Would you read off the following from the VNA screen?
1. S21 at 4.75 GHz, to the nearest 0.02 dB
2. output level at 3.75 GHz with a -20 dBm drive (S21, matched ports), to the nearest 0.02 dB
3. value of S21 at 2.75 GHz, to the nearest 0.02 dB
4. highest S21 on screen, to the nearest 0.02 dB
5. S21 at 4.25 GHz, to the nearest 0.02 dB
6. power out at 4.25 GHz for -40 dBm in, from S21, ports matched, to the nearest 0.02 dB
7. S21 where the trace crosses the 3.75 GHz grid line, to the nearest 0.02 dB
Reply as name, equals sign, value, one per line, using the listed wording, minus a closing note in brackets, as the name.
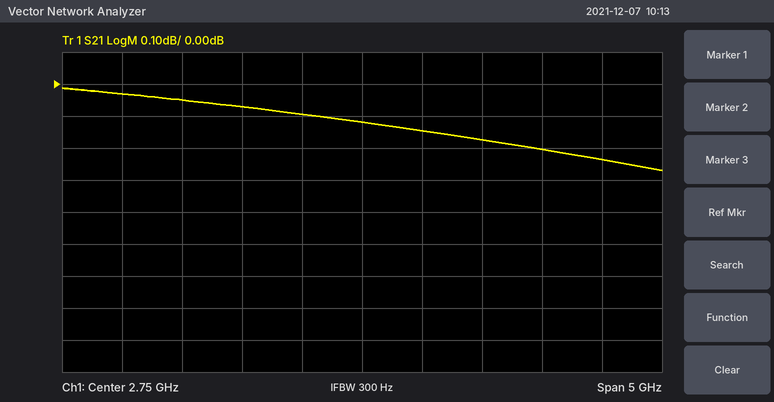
S21 at 4.75 GHz, to the nearest 0.02 dB = -0.24 dB
output level at 3.75 GHz with a -20 dBm drive (S21, matched ports), to the nearest 0.02 dB = -20.18 dBm
value of S21 at 2.75 GHz, to the nearest 0.02 dB = -0.12 dB
highest S21 on screen, to the nearest 0.02 dB = -0.02 dB
S21 at 4.25 GHz, to the nearest 0.02 dB = -0.20 dB
power out at 4.25 GHz for -40 dBm in, from S21, ports matched, to the nearest 0.02 dB = -40.20 dBm
S21 where the trace crosses the 3.75 GHz grid line, to the nearest 0.02 dB = -0.18 dB
